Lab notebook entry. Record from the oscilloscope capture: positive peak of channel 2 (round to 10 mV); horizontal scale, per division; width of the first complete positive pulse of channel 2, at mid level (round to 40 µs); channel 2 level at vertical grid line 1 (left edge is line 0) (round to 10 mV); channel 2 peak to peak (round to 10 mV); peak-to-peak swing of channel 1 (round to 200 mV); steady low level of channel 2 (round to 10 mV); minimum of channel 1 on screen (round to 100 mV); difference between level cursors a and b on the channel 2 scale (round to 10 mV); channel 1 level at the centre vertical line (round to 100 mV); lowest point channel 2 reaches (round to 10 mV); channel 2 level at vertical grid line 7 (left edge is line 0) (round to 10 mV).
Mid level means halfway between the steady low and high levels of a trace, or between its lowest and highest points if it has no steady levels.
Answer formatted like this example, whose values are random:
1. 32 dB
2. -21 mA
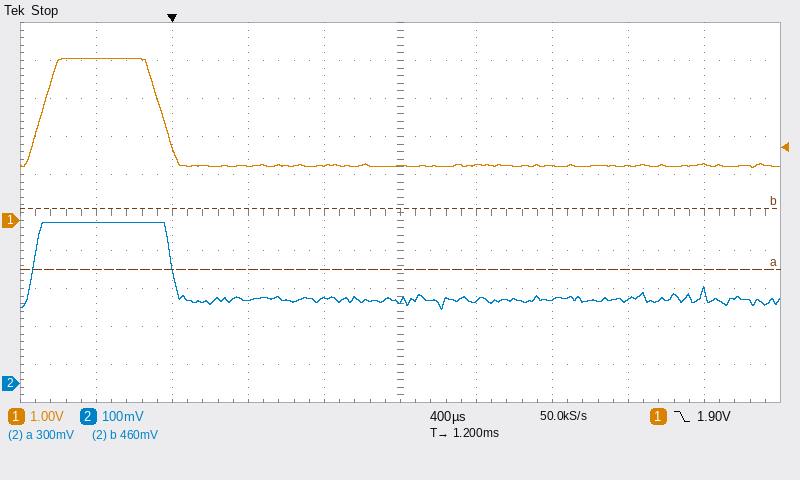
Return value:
1. 420 mV
2. 400 µs
3. 720 µs
4. 420 mV
5. 230 mV
6. 2.8 V
7. 220 mV
8. 1.4 V
9. 160 mV
10. 1.4 V
11. 190 mV
12. 220 mV
